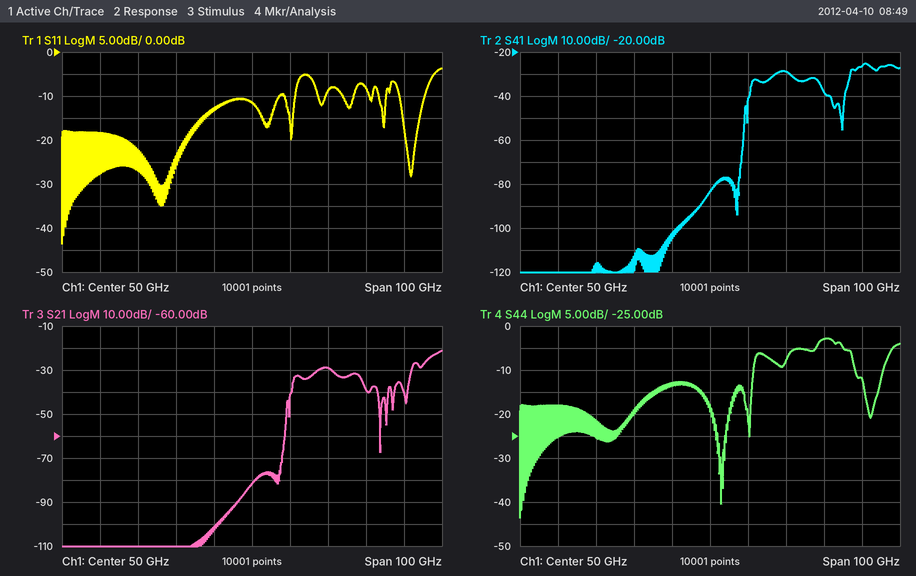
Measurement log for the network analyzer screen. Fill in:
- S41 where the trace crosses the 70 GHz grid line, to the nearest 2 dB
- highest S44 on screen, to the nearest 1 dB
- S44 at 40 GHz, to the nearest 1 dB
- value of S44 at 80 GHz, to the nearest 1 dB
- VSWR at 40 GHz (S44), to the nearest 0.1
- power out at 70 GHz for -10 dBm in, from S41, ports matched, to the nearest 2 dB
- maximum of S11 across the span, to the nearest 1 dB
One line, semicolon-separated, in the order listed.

-28 dB; -3 dB; -13 dB; -3 dB; 1.6; -38 dBm; -4 dB
